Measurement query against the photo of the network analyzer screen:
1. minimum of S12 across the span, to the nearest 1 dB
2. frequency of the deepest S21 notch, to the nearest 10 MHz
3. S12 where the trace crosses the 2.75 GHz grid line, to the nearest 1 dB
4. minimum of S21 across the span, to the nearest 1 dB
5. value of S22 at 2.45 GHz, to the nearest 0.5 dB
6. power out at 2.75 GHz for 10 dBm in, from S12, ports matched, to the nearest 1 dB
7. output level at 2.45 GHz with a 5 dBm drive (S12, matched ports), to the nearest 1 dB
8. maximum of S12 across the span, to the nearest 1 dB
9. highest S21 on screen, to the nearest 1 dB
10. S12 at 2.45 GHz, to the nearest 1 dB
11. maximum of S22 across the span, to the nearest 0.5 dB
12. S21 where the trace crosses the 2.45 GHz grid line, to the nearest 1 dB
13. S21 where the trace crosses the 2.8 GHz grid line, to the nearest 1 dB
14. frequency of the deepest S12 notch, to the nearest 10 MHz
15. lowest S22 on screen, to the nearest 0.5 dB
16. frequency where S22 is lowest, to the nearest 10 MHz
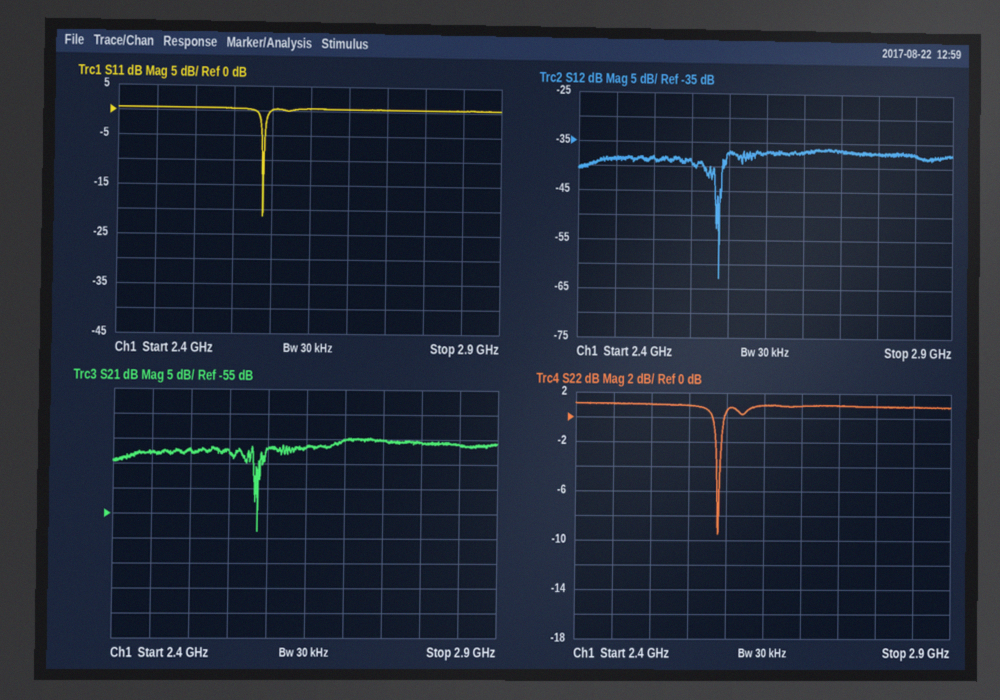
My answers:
-63 dB
2.59 GHz
-37 dB
-59 dB
1.0 dB
-27 dBm
-34 dBm
-36 dB
-40 dB
-39 dB
1.0 dB
-43 dB
-41 dB
2.59 GHz
-9.5 dB
2.59 GHz
